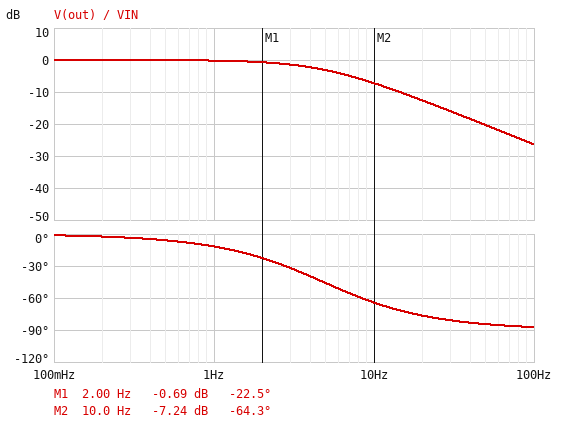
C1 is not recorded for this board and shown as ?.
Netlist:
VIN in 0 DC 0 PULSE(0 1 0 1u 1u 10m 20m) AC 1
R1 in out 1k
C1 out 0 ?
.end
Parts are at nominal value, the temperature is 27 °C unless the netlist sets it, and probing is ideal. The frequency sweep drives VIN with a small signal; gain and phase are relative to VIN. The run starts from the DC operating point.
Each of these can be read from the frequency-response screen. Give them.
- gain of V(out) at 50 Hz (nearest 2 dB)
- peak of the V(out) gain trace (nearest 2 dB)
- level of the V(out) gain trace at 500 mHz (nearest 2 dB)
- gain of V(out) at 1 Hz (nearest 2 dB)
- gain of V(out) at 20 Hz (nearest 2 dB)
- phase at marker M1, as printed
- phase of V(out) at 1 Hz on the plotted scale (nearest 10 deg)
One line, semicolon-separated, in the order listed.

-20 dB; 0 dB; 0 dB; 0 dB; -12 dB; -22.5 deg; -10 deg
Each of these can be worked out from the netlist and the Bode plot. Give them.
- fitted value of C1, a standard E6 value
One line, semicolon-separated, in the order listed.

33 µF
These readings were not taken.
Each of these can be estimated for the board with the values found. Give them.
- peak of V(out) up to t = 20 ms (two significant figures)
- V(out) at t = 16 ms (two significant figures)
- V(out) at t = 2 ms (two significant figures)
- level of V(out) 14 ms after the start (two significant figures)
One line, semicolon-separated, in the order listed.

260 mV; 220 mV; 59 mV; 230 mV
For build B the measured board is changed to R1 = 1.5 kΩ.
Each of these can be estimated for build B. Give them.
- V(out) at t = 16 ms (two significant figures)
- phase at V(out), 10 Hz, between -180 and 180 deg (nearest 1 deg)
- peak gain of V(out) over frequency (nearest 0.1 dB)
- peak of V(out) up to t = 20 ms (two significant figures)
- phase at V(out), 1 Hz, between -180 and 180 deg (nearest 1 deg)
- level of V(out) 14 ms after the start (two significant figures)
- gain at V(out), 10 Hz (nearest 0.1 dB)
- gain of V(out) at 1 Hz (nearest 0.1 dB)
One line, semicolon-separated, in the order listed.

160 mV; -72 deg; 0 dB; 180 mV; -17 deg; 170 mV; -10.3 dB; -0.4 dB
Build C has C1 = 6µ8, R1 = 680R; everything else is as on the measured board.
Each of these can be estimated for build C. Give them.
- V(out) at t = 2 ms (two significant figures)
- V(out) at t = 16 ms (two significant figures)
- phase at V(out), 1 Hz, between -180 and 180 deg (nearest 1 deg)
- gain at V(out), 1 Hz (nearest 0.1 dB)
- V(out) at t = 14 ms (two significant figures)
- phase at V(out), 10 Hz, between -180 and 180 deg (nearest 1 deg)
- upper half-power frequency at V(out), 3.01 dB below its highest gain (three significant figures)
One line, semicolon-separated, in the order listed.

350 mV; 240 mV; -2 deg; 0 dB; 370 mV; -16 deg; 34.4 Hz
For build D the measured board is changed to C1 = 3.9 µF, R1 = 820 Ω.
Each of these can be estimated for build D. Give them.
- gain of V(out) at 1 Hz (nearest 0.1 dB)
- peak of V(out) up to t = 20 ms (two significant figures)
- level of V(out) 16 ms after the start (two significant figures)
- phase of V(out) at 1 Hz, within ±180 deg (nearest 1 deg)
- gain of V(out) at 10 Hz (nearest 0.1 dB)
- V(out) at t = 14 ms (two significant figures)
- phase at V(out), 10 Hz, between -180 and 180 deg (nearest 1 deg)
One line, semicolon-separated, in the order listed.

0 dB; 960 mV; 150 mV; -1 deg; -0.2 dB; 270 mV; -11 deg
